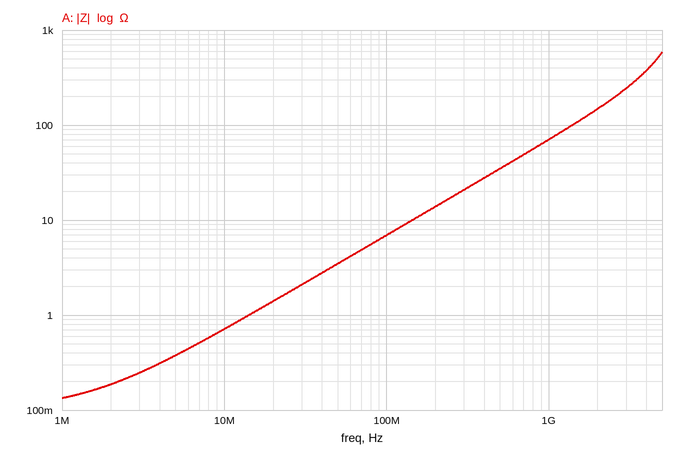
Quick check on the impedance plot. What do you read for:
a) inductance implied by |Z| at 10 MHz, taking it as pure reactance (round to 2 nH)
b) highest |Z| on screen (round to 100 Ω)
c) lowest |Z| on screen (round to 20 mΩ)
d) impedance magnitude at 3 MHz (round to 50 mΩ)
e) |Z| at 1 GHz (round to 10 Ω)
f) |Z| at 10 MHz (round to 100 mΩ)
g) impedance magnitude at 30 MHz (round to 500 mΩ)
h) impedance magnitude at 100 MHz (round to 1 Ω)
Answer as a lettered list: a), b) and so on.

a) 12 nH
b) 600 Ω
c) 140 mΩ
d) 250 mΩ
e) 70 Ω
f) 700 mΩ
g) 2.0 Ω
h) 7 Ω
